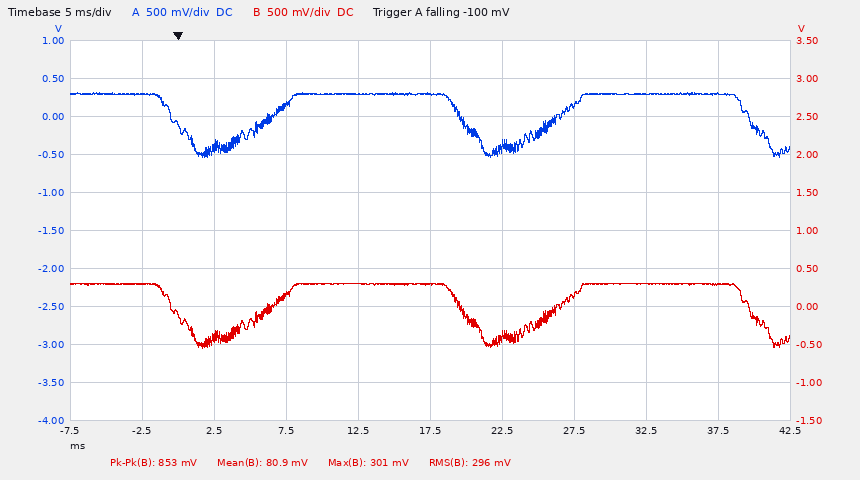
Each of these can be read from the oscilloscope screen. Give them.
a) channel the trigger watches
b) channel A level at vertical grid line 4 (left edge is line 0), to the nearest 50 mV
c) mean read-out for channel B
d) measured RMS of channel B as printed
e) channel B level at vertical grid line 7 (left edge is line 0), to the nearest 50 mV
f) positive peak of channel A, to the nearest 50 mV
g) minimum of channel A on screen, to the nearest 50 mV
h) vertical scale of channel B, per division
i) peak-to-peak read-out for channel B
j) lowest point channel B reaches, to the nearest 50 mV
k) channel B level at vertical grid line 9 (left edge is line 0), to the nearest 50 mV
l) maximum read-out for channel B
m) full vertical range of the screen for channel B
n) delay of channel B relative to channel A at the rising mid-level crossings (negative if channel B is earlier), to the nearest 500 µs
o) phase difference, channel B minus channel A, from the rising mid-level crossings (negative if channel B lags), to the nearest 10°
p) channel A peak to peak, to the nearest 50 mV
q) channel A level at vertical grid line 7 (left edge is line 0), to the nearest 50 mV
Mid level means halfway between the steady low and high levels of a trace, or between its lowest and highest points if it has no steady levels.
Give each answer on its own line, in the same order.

channel A
300 mV
80.9 mV
296 mV
150 mV
300 mV
-550 mV
500 mV
853 mV
-550 mV
300 mV
301 mV
5 V
0.0 ms
0°
850 mV
150 mV
